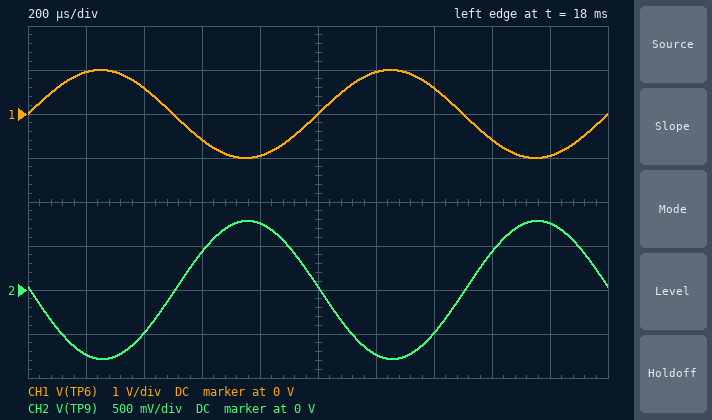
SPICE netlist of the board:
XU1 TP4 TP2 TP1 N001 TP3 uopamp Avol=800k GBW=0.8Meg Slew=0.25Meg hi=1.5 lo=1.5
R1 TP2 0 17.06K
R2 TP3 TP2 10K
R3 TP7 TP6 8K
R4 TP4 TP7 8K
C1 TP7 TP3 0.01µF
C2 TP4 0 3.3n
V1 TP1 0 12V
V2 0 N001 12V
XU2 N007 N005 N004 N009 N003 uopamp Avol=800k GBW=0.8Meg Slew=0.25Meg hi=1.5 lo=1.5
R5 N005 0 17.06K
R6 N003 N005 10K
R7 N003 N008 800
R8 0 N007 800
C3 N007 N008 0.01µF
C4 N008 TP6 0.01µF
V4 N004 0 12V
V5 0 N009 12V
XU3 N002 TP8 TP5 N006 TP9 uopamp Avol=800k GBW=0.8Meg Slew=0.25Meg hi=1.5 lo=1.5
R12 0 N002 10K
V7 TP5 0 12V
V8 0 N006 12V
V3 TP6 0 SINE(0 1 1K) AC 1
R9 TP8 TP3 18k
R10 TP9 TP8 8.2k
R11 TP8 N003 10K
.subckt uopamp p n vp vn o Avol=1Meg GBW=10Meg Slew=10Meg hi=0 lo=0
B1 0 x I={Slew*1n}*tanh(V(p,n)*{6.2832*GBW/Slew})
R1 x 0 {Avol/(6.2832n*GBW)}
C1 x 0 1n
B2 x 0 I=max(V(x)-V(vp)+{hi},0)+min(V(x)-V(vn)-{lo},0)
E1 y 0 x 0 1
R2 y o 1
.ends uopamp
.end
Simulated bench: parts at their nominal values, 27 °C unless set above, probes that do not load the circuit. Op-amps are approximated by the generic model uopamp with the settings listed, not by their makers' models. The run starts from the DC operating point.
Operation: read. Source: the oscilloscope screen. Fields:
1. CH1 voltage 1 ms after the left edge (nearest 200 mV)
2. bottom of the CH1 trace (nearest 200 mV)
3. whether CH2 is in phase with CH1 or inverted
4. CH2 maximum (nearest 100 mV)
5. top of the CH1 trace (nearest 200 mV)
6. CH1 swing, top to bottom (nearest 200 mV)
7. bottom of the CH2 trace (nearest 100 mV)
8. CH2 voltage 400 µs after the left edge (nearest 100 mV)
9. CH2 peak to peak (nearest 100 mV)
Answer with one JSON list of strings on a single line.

["0 V", "-1.0 V", "inverted", "800 mV", "1.0 V", "2.0 V", "-800 mV", "-500 mV", "1.6 V"]
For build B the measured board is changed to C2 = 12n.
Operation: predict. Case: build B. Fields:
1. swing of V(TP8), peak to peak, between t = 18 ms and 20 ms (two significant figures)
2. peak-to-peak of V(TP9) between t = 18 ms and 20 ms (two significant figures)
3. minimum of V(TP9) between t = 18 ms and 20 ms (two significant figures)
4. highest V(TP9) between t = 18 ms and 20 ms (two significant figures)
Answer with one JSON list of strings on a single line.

["1.6 mV", "1.3 V", "-630 mV", "630 mV"]
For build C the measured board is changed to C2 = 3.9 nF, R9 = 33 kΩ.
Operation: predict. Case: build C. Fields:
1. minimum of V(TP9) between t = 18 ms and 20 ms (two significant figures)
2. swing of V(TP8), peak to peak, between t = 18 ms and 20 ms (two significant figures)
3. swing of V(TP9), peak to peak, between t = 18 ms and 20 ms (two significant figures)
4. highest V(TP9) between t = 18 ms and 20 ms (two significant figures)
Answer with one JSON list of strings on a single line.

["-430 mV", "1.1 mV", "860 mV", "430 mV"]
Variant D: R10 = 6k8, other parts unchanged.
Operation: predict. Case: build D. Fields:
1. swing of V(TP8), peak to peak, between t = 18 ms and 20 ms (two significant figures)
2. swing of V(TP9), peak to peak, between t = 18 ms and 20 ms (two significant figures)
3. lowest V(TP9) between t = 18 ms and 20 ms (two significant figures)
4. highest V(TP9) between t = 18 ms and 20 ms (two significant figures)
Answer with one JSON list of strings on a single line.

["1.6 mV", "1.3 V", "-650 mV", "650 mV"]
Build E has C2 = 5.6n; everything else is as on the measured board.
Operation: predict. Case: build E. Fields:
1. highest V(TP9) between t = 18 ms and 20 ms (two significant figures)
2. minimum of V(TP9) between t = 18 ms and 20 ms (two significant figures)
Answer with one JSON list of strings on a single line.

["800 mV", "-800 mV"]
